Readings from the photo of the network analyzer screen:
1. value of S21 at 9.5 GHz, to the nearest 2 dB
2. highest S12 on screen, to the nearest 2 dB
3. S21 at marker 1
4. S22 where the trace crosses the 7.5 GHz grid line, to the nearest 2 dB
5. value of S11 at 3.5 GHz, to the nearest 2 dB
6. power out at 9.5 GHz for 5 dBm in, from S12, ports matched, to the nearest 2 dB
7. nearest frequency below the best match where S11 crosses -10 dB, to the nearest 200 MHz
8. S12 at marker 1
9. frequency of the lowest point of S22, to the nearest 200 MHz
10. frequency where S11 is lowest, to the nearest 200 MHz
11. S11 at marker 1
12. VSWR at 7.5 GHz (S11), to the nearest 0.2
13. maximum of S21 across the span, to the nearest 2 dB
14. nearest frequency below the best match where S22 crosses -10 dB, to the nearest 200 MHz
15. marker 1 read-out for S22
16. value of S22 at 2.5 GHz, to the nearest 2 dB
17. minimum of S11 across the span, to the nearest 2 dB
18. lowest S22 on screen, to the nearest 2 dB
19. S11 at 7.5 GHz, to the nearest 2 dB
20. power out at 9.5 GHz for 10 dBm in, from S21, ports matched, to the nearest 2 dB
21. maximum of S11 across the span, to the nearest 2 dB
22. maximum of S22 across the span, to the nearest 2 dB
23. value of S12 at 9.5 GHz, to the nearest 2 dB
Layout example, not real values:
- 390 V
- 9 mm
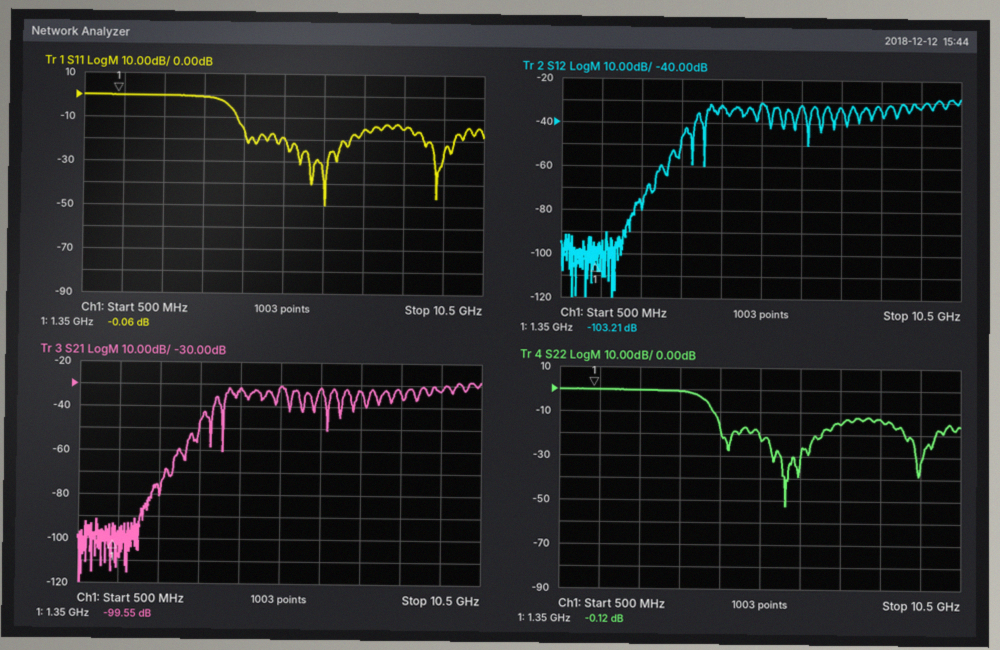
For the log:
- -32 dB
- -28 dB
- -99.55 dB
- -16 dB
- 0 dB
- -28 dBm
- 4.4 GHz
- -103.21 dB
- 6.2 GHz
- 6.6 GHz
- -0.06 dB
- 1.4
- -28 dB
- 4.4 GHz
- -0.12 dB
- 0 dB
- -50 dB
- -52 dB
- -16 dB
- -22 dBm
- 0 dB
- 0 dB
- -32 dB
